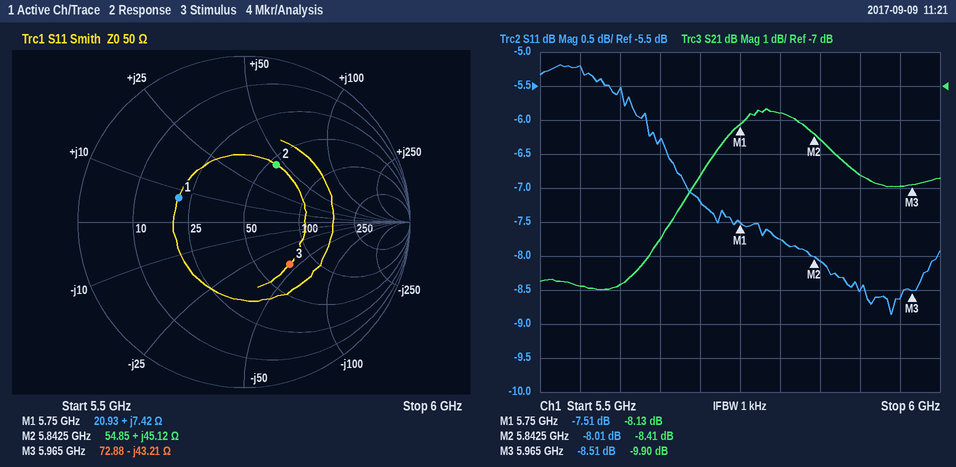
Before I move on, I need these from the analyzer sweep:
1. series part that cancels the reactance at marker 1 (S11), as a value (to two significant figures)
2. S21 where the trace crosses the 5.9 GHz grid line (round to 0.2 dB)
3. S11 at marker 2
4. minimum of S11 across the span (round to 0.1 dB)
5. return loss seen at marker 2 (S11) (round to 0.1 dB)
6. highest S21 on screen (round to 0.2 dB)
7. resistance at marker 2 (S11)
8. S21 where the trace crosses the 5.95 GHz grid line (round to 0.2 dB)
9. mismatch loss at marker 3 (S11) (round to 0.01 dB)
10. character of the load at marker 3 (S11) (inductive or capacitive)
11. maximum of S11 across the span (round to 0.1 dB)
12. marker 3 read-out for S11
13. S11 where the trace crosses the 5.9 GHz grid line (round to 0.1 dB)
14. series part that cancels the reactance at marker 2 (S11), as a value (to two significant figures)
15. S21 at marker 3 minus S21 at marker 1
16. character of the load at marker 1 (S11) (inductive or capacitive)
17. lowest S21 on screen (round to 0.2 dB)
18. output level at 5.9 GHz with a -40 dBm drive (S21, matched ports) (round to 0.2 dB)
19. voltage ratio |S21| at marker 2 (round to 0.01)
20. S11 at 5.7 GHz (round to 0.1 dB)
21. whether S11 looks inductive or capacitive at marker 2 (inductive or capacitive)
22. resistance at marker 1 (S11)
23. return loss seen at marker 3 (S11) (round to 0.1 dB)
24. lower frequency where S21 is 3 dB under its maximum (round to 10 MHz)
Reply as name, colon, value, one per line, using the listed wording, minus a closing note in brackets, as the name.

series part that cancels the reactance at marker 1 (S11), as a value: 3.7 pF
S21 where the trace crosses the 5.9 GHz grid line: -9.6 dB
S11 at marker 2: -8.01 dB
minimum of S11 across the span: -8.9 dB
return loss seen at marker 2 (S11): 8.0 dB
highest S21 on screen: -7.6 dB
resistance at marker 2: 54.85 Ω
S21 where the trace crosses the 5.95 GHz grid line: -10.0 dB
mismatch loss at marker 3 (S11): 0.66 dB
character of the load at marker 3 (S11): capacitive
maximum of S11 across the span: -5.2 dB
marker 3 read-out for S11: -8.51 dB
S11 where the trace crosses the 5.9 GHz grid line: -8.5 dB
series part that cancels the reactance at marker 2 (S11), as a value: 600 fF
S21 at marker 3 minus S21 at marker 1: -1.77 dB
character of the load at marker 1 (S11): inductive
lowest S21 on screen: -13.0 dB
output level at 5.9 GHz with a -40 dBm drive (S21, matched ports): -49.6 dBm
voltage ratio |S21| at marker 2: 0.38
S11 at 5.7 GHz: -7.2 dB
whether S11 looks inductive or capacitive at marker 2: inductive
resistance at marker 1: 20.93 Ω
return loss seen at marker 3 (S11): 8.5 dB
lower frequency where S21 is 3 dB under its maximum: 5.67 GHz
